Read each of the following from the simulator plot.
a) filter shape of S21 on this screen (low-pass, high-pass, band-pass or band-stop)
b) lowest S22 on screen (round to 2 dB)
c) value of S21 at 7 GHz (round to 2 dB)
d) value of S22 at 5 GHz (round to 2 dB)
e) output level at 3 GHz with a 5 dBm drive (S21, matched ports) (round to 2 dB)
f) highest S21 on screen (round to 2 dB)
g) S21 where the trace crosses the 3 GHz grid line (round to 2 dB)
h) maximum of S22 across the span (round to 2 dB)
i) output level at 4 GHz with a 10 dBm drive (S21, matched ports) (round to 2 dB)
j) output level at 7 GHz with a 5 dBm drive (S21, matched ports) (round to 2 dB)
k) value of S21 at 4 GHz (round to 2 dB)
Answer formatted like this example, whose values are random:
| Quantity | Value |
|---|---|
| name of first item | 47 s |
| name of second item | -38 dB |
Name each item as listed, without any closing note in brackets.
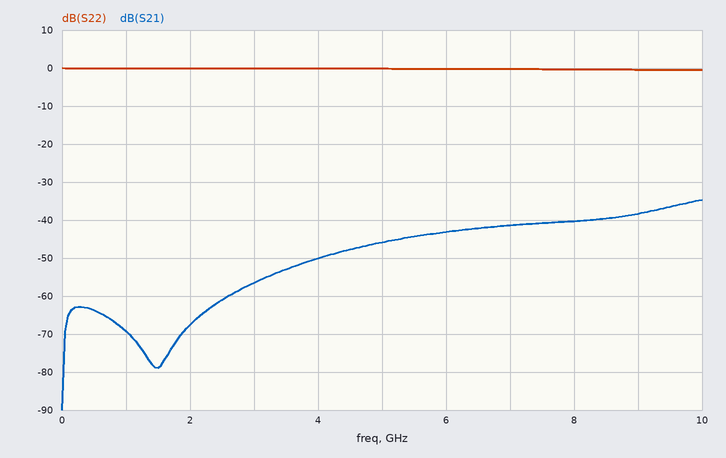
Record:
| Quantity | Value |
|---|---|
| filter shape of S21 on this screen | high-pass |
| lowest S22 on screen | 0 dB |
| value of S21 at 7 GHz | -42 dB |
| value of S22 at 5 GHz | 0 dB |
| output level at 3 GHz with a 5 dBm drive (S21, matched ports) | -52 dBm |
| highest S21 on screen | -34 dB |
| S21 where the trace crosses the 3 GHz grid line | -56 dB |
| maximum of S22 across the span | 0 dB |
| output level at 4 GHz with a 10 dBm drive (S21, matched ports) | -40 dBm |
| output level at 7 GHz with a 5 dBm drive (S21, matched ports) | -36 dBm |
| value of S21 at 4 GHz | -50 dB |
